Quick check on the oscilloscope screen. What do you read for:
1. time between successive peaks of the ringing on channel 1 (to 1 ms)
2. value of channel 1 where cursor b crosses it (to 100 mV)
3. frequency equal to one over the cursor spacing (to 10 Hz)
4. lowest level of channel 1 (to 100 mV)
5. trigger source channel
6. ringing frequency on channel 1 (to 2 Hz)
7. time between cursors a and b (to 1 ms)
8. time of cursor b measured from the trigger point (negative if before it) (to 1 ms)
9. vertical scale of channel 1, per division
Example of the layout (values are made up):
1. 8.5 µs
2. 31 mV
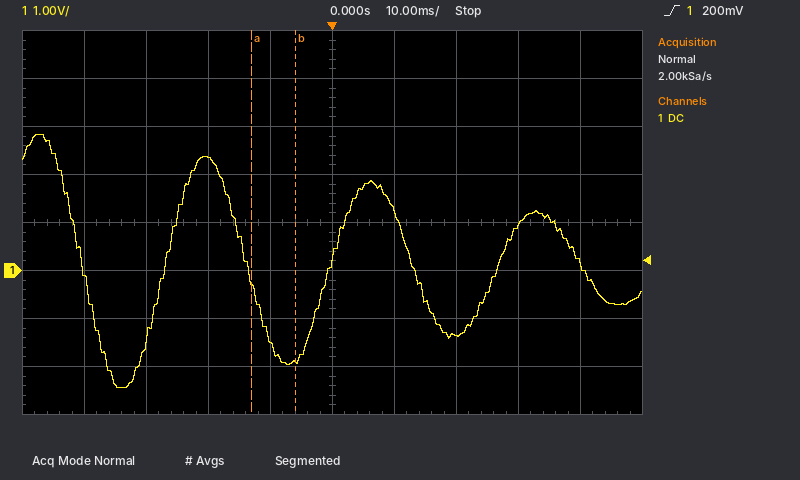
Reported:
1. 27 ms
2. -1.9 V
3. 140 Hz
4. -2.4 V
5. channel 1
6. 38 Hz
7. 7 ms
8. -6 ms
9. 1 V
